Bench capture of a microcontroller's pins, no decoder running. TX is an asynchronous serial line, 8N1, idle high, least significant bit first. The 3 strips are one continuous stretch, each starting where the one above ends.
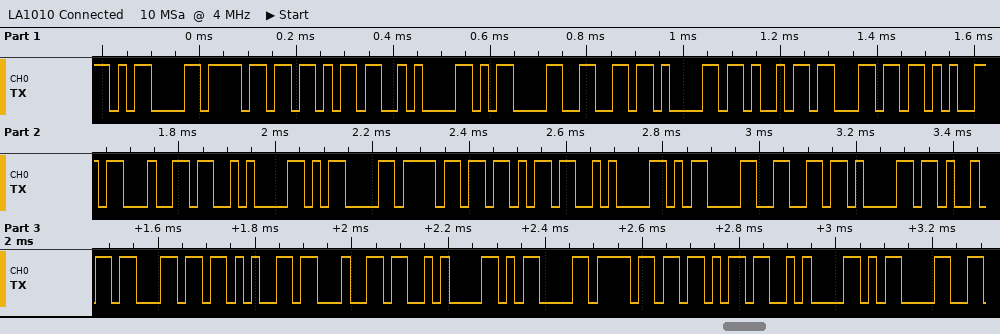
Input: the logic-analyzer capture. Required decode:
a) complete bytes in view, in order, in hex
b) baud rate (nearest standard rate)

0D 6F 6B 0A 0D 66 61 69 6C 65 64 0A 0D 6F 6B 0A 0D 66 61 69 6C 65 64 0A 0D 6F 6B 0A 0D
57600 baud
